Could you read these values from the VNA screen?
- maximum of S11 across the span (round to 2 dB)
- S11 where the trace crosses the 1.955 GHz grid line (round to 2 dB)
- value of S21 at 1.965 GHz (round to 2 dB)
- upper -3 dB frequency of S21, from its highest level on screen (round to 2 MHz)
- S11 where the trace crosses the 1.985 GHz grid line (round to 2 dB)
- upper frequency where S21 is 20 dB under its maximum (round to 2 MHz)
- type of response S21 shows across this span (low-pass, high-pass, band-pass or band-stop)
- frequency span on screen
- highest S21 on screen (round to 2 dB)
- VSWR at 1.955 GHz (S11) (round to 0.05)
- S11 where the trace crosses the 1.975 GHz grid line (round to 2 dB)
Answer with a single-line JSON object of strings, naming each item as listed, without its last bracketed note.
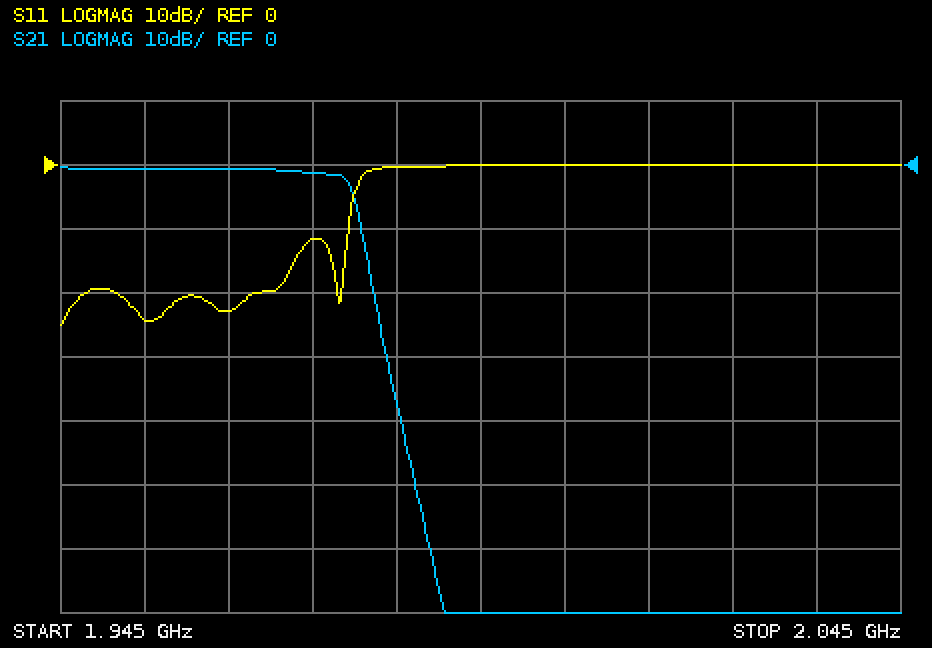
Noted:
{"maximum of S11 across the span": "0 dB", "S11 where the trace crosses the 1.955 GHz grid line": "-24 dB", "value of S21 at 1.965 GHz": "0 dB", "upper -3 dB frequency of S21, from its highest level on screen": "1.980 GHz", "S11 where the trace crosses the 1.985 GHz grid line": "0 dB", "upper frequency where S21 is 20 dB under its maximum": "1.982 GHz", "type of response S21 shows across this span": "low-pass", "frequency span on screen": "100 MHz", "highest S21 on screen": "0 dB", "VSWR at 1.955 GHz (S11)": "1.15", "S11 where the trace crosses the 1.975 GHz grid line": "-12 dB"}
